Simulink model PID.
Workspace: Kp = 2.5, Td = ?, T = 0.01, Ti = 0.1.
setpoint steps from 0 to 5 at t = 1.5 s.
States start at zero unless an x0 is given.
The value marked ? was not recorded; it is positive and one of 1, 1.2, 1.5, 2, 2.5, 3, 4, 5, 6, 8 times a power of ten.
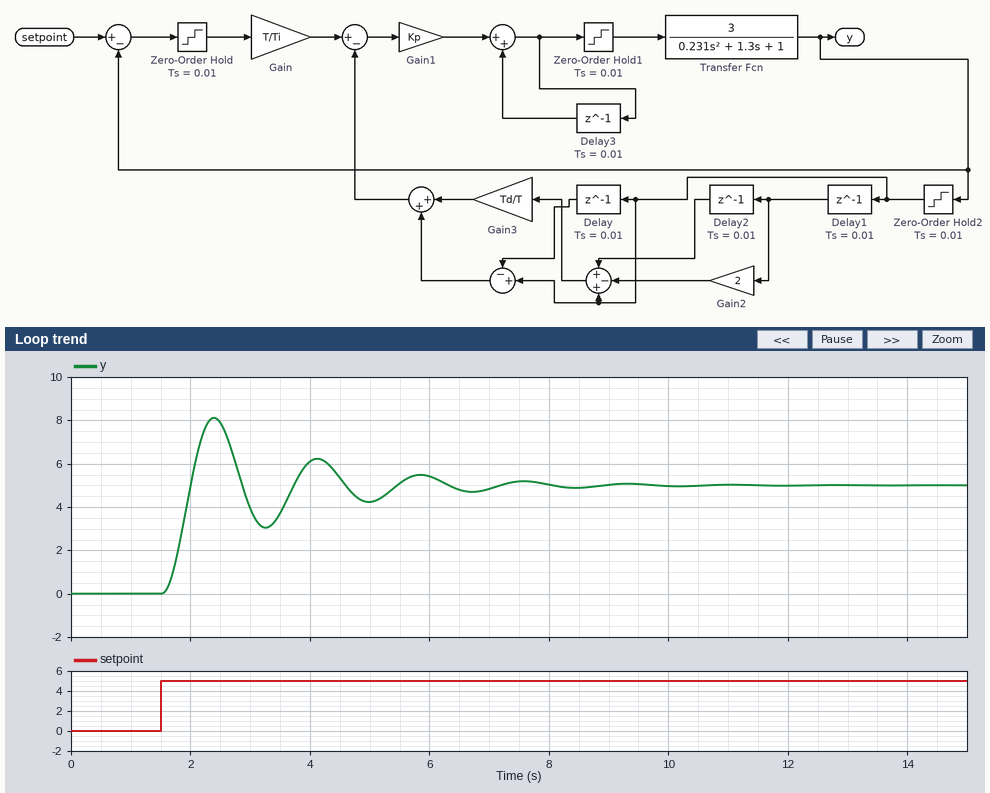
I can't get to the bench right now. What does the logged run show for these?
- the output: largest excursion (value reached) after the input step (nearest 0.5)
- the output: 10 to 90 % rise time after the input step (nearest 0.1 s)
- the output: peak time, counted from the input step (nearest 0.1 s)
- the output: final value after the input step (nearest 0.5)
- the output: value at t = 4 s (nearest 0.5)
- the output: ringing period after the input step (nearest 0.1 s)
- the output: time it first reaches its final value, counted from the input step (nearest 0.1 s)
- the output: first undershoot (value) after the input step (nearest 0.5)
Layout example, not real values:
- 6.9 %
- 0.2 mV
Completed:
- 8.0
- 0.3 s
- 0.9 s
- 5.0
- 6.0
- 1.7 s
- 0.5 s
- 3.0
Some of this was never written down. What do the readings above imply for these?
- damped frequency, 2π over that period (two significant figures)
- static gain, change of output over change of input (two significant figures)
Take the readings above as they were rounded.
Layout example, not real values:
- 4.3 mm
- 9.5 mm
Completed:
- 3.7 rad/s
- 1.0
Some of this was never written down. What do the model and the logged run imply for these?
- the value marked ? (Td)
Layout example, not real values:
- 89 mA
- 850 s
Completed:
- 0.6
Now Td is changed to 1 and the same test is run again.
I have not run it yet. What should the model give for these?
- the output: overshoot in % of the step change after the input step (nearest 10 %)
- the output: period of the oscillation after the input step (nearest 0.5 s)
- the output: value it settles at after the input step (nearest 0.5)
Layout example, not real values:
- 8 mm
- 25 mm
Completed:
- 60 %
- 2.0 s
- 5.0
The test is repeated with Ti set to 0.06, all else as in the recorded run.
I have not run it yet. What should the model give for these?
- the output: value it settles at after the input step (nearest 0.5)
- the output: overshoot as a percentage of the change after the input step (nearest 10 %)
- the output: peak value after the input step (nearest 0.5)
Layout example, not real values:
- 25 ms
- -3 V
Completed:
- 5.0
- 80 %
- 9.0
